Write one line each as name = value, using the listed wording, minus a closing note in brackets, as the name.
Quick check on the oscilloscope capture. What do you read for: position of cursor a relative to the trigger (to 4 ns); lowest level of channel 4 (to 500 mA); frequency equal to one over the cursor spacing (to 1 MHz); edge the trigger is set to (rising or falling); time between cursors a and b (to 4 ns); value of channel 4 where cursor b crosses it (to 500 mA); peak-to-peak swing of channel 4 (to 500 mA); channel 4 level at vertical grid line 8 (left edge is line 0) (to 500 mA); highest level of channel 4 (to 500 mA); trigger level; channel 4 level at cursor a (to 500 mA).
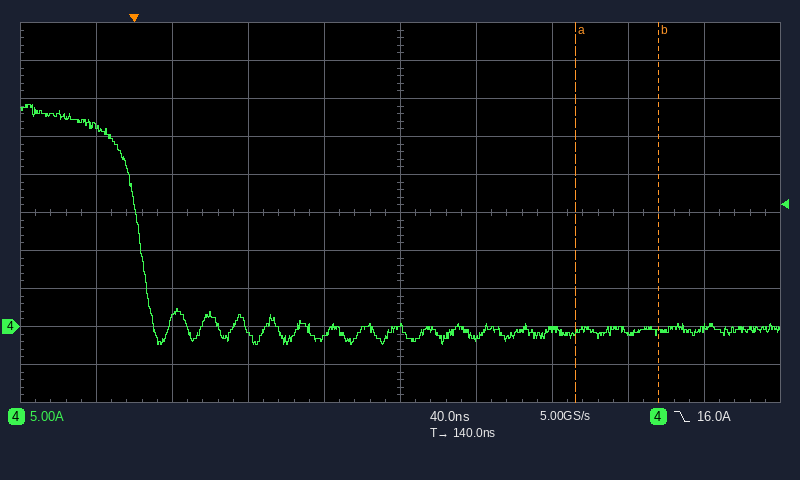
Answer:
position of cursor a relative to the trigger = +232 ns
lowest level of channel 4 = -2.5 A
frequency equal to one over the cursor spacing = 23 MHz
edge the trigger is set to = falling
time between cursors a and b = 44 ns
value of channel 4 where cursor b crosses it = -1.0 A
peak-to-peak swing of channel 4 = 31.5 A
channel 4 level at vertical grid line 8 (left edge is line 0) = -1.0 A
highest level of channel 4 = 29.0 A
trigger level = 16.0 A
channel 4 level at cursor a = -1.0 A
